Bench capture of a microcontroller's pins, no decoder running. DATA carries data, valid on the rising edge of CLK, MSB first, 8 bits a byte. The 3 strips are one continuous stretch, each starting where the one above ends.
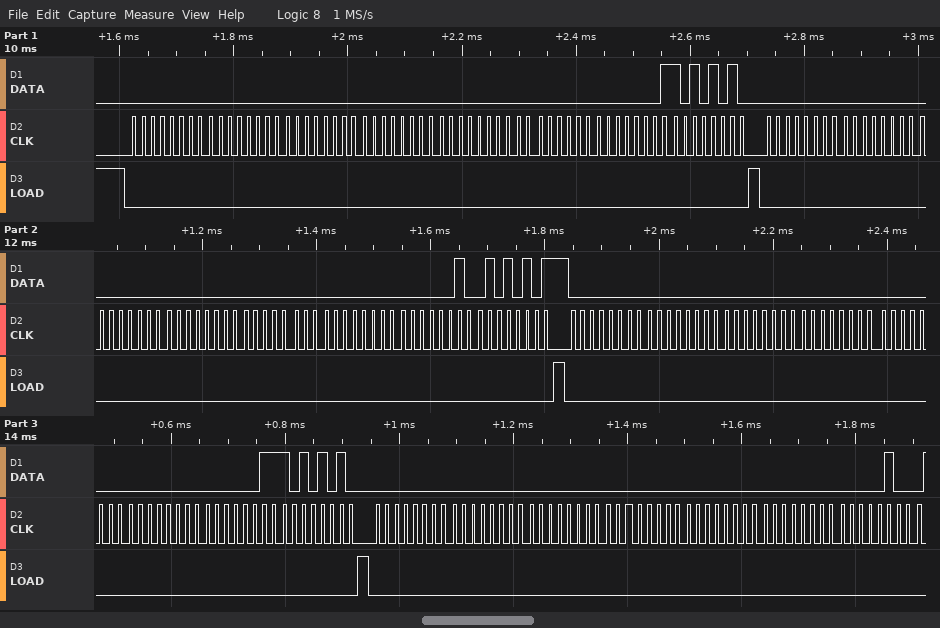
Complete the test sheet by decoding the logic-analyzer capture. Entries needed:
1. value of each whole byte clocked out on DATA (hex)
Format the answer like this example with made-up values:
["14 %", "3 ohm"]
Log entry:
["00 00 00 00 00 00 01 AA 00 00 00 00 00 00 02 55 00 00 00 00 00 00 03 AA 00 00 00 00 00 00 04"]
